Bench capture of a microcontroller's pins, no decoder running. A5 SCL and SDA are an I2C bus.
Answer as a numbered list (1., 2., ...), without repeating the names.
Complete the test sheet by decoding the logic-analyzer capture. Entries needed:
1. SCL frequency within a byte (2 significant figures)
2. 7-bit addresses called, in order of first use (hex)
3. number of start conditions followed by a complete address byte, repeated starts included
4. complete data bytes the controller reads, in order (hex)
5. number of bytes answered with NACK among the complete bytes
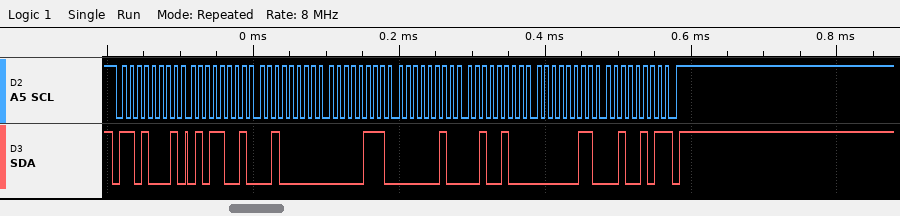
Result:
1. 100 kHz
2. 0x68
3. 1
4. 59 20 07 02 24 03 25
5. 1
